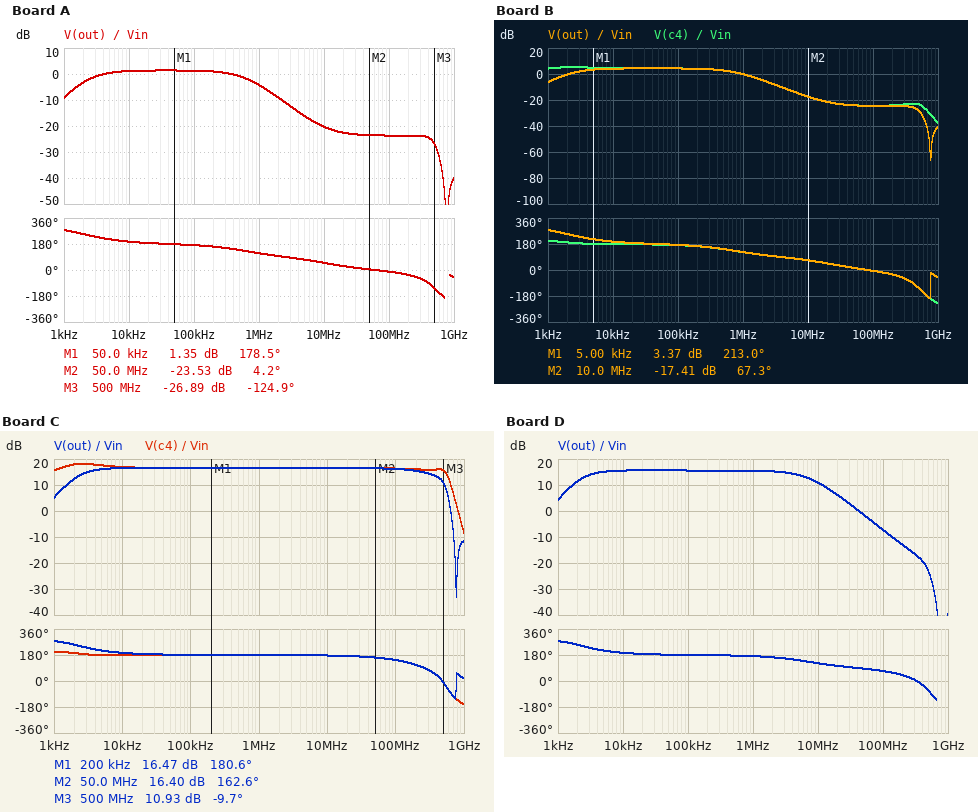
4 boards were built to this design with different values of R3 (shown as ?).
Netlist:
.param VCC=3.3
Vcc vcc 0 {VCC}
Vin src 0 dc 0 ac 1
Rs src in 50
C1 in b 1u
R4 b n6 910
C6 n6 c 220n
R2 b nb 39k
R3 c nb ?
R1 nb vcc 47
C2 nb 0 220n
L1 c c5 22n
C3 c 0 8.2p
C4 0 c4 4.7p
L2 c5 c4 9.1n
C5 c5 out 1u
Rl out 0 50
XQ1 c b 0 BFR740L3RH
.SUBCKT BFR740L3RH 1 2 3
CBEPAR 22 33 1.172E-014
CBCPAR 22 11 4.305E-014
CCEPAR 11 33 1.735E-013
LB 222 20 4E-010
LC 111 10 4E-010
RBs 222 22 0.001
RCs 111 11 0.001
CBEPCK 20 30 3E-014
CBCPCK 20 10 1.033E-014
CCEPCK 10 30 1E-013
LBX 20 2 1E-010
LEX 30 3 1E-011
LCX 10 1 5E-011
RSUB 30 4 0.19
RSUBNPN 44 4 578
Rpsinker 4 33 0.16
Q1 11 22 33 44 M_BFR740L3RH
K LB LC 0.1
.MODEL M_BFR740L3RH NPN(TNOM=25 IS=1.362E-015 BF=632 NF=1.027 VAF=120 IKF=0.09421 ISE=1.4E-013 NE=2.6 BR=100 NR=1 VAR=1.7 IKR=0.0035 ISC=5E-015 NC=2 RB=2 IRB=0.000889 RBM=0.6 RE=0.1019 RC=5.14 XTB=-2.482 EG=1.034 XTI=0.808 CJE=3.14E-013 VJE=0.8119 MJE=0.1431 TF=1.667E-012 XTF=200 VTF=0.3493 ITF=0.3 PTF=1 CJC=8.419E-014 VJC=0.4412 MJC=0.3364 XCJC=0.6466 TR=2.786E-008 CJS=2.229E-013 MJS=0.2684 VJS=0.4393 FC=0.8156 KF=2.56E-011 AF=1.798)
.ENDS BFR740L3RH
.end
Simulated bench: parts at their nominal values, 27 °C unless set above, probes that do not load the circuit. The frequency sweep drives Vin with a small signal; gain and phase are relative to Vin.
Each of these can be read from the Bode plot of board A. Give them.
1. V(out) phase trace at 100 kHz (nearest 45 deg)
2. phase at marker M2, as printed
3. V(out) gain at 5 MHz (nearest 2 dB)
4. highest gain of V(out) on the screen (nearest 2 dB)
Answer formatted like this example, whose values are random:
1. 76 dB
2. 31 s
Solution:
1. 180 deg
2. 4.2 deg
3. -16 dB
4. 2 dB
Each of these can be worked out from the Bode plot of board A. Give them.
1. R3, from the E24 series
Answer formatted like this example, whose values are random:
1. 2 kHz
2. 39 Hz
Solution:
1. 430 Ω
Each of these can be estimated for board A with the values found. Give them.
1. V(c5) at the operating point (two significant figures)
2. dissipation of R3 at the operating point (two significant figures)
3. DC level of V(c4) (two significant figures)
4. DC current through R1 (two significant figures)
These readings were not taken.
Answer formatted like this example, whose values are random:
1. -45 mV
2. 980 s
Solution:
1. 120 mV
2. 19 mW
3. 120 mV
4. 6.7 mA
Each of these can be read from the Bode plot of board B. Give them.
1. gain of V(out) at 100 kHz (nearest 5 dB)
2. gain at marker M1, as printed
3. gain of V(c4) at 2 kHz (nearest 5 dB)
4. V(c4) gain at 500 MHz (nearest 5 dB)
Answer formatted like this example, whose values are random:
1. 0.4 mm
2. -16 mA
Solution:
1. 5 dB
2. 3.37 dB
3. 5 dB
4. -25 dB
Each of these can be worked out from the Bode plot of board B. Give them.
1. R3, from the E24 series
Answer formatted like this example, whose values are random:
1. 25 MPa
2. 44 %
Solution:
1. 330 Ω
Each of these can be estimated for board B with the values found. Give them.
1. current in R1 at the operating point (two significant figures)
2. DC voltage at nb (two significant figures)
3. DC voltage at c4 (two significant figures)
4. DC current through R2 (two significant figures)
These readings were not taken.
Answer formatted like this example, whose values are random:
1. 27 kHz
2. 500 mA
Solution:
1. 8.4 mA
2. 2.9 V
3. 140 mV
4. 54 µA
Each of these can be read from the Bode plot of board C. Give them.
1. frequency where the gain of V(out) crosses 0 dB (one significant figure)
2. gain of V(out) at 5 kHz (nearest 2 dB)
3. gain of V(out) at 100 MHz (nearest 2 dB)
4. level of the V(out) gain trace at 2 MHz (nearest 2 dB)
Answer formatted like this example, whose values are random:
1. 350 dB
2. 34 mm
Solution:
1. 600 MHz
2. 16 dB
3. 16 dB
4. 16 dB
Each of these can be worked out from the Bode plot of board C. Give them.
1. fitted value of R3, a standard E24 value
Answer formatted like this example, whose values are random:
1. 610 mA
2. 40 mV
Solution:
1. 180 Ω
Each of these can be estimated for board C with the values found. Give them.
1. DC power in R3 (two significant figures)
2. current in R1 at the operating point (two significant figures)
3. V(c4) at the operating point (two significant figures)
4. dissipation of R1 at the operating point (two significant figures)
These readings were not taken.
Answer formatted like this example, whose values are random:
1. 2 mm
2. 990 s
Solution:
1. 28 mW
2. 13 mA
3. 460 mV
4. 7.4 mW
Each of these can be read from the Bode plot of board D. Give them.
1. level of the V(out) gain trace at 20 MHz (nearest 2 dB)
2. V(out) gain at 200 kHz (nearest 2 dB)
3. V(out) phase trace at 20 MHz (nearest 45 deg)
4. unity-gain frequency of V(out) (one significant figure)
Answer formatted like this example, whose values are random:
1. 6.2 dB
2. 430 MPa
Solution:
1. 6 dB
2. 16 dB
3. 90 deg
4. 40 MHz
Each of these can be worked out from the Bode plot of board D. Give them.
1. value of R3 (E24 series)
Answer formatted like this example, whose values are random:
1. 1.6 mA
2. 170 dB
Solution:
1. 200 Ω
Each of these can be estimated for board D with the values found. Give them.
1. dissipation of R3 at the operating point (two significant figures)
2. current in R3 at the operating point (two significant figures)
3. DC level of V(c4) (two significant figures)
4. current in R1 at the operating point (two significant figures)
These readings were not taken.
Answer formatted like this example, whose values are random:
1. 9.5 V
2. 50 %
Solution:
1. 30 mW
2. 12 mA
3. 260 mV
4. 12 mA
